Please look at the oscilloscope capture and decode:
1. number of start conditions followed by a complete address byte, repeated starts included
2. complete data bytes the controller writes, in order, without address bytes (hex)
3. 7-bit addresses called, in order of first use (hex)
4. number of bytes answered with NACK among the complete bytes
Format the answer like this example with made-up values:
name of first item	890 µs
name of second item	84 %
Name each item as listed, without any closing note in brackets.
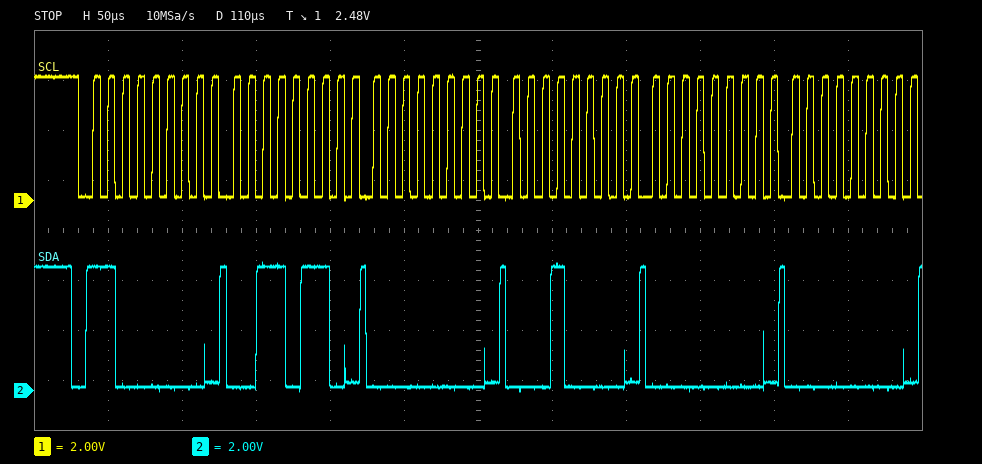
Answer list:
number of start conditions followed by a complete address byte, repeated starts included	1
complete data bytes the controller writes, in order, without address bytes	36 00 10 00 00
7-bit addresses called, in order of first use	0x60
number of bytes answered with NACK among the complete bytes	0
